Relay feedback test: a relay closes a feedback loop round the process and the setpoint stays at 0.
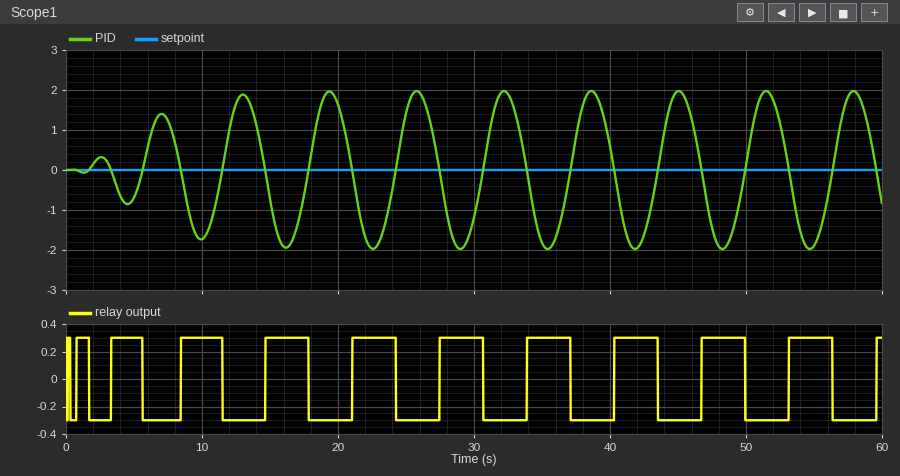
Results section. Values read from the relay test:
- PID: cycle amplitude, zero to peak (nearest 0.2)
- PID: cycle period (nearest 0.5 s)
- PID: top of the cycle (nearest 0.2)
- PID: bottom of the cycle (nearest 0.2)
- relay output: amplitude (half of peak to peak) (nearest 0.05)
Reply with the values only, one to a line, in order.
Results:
2.0
6.5 s
2.0
-2.0
0.30
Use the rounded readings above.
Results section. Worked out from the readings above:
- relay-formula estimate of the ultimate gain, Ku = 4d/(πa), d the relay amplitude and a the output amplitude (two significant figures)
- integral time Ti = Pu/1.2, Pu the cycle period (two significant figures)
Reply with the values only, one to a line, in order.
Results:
0.19
5.4 s
